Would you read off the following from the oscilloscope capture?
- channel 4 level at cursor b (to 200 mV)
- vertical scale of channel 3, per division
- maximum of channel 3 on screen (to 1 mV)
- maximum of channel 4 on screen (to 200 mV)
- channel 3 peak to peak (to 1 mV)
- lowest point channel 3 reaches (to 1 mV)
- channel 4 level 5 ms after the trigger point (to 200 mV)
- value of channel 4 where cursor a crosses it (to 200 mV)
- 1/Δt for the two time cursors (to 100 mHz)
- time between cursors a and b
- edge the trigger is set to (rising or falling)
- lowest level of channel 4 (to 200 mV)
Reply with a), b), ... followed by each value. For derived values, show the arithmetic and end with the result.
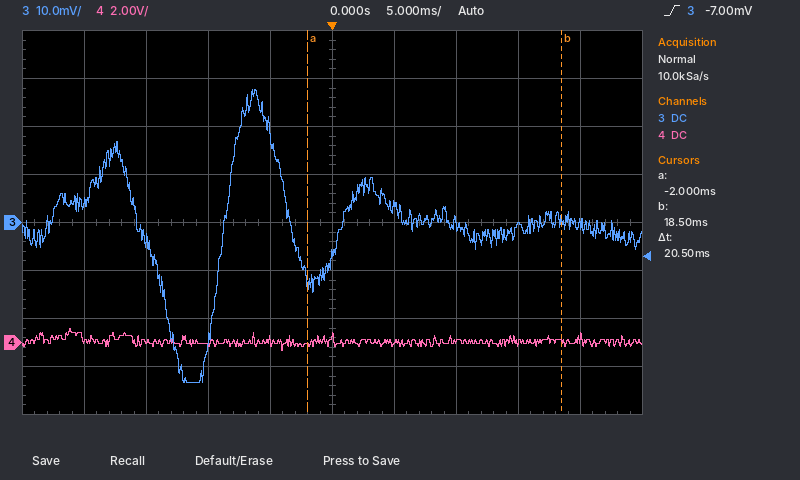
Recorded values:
a) 0.0 V
b) 10 mV
c) 28 mV
d) 600 mV
e) 28 mV − (-33 mV) = 61 mV
f) -33 mV
g) 0.0 V
h) 0.0 V
i) 1 / 20.5 ms ≈ 48.8 Hz
j) 20.5 ms
k) rising
l) -400 mV
